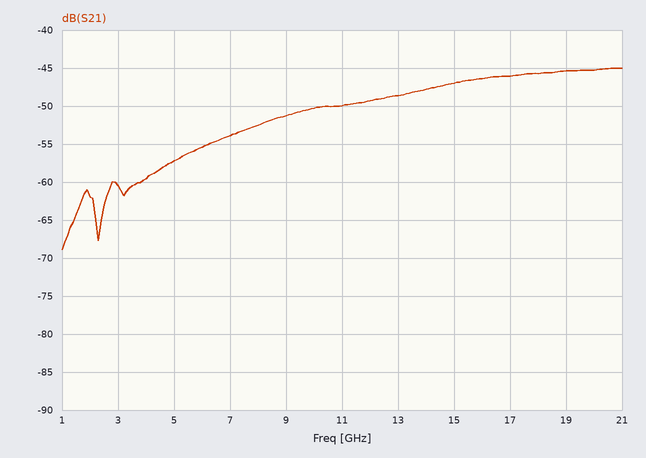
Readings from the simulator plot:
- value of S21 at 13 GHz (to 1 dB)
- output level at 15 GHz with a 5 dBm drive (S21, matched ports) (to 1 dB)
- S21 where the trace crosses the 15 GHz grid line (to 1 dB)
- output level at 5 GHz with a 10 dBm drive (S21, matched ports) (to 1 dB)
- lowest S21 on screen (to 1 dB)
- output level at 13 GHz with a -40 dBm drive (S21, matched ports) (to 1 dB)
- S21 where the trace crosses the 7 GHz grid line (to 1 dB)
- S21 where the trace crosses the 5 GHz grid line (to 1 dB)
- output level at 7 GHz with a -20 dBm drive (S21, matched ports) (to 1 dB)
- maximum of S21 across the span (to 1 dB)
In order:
-49 dB
-42 dBm
-47 dB
-47 dBm
-69 dB
-89 dBm
-54 dB
-57 dB
-74 dBm
-45 dB
